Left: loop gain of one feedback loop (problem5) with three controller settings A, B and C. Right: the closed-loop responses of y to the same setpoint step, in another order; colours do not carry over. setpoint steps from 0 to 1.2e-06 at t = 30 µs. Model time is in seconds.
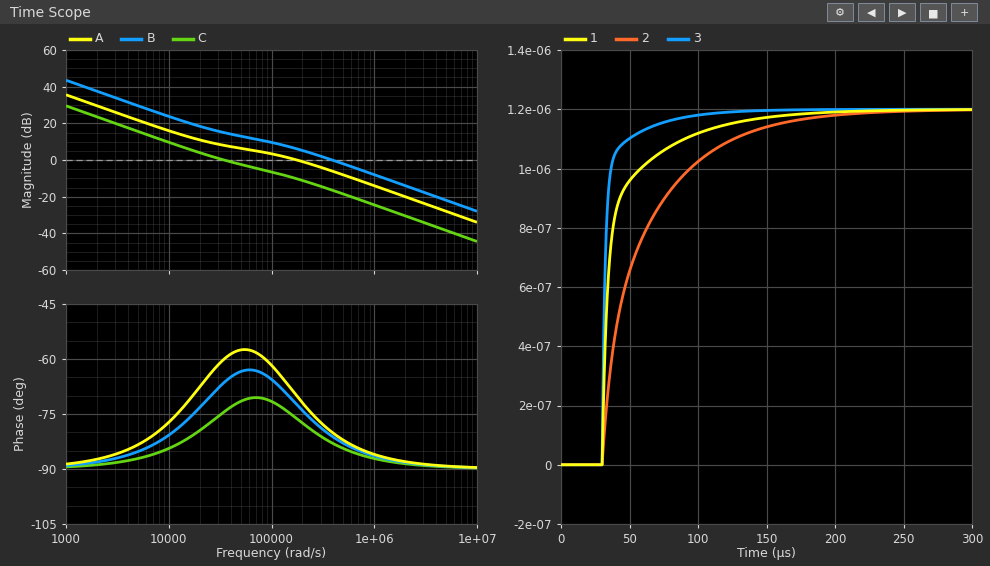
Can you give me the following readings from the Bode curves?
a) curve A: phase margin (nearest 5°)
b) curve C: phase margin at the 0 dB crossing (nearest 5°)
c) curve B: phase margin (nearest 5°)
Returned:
110°
105°
100°
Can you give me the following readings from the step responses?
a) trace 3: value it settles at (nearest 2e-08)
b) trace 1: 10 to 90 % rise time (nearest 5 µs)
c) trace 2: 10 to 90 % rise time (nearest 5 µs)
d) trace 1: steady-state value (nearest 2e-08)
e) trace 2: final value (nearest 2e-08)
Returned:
0.00000120
50 µs
85 µs
0.00000120
0.00000120
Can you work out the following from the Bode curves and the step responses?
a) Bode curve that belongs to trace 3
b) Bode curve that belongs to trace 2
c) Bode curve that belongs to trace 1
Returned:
B
C
A
